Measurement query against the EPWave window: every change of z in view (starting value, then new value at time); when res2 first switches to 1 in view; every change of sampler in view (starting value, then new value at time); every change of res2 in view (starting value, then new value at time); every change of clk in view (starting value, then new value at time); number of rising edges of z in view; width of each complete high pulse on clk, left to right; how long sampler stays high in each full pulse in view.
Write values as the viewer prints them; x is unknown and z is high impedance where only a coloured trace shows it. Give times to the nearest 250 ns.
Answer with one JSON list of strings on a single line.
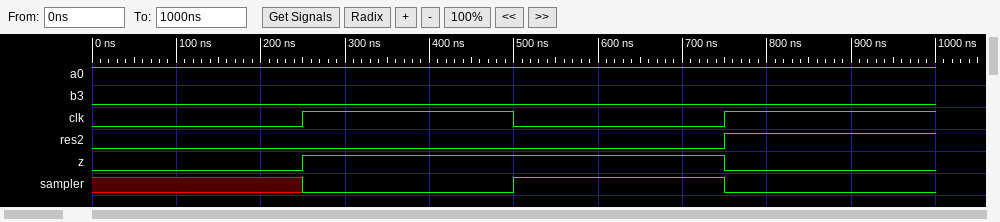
["0, 1 at 250 ns, 0 at 750 ns", "750 ns", "x, 0 at 250 ns, 1 at 500 ns, 0 at 750 ns", "0, 1 at 750 ns", "0, 1 at 250 ns, 0 at 500 ns, 1 at 750 ns", "1", "250 ns", "250 ns"]
